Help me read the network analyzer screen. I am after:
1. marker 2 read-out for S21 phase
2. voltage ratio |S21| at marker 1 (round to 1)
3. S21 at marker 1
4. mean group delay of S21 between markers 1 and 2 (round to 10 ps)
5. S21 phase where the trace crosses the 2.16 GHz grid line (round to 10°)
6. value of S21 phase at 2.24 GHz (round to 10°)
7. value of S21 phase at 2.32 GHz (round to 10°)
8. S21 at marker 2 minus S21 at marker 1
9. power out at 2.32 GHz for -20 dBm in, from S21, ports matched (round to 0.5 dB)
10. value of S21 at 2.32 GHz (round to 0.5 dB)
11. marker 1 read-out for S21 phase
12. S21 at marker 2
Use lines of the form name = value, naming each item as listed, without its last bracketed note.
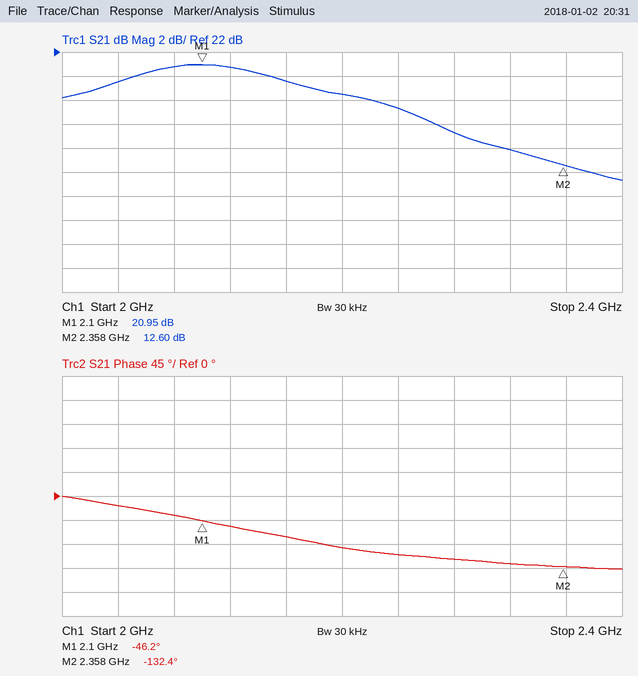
marker 2 read-out for S21 phase = -132.4°
voltage ratio |S21| at marker 1 = 11
S21 at marker 1 = 20.95 dB
mean group delay of S21 between markers 1 and 2 = 930 ps
S21 phase where the trace crosses the 2.16 GHz grid line = -80°
value of S21 phase at 2.24 GHz = -110°
value of S21 phase at 2.32 GHz = -130°
S21 at marker 2 minus S21 at marker 1 = -8.35 dB
power out at 2.32 GHz for -20 dBm in, from S21, ports matched = -6.0 dBm
value of S21 at 2.32 GHz = 14.0 dB
marker 1 read-out for S21 phase = -46.2°
S21 at marker 2 = 12.60 dB
